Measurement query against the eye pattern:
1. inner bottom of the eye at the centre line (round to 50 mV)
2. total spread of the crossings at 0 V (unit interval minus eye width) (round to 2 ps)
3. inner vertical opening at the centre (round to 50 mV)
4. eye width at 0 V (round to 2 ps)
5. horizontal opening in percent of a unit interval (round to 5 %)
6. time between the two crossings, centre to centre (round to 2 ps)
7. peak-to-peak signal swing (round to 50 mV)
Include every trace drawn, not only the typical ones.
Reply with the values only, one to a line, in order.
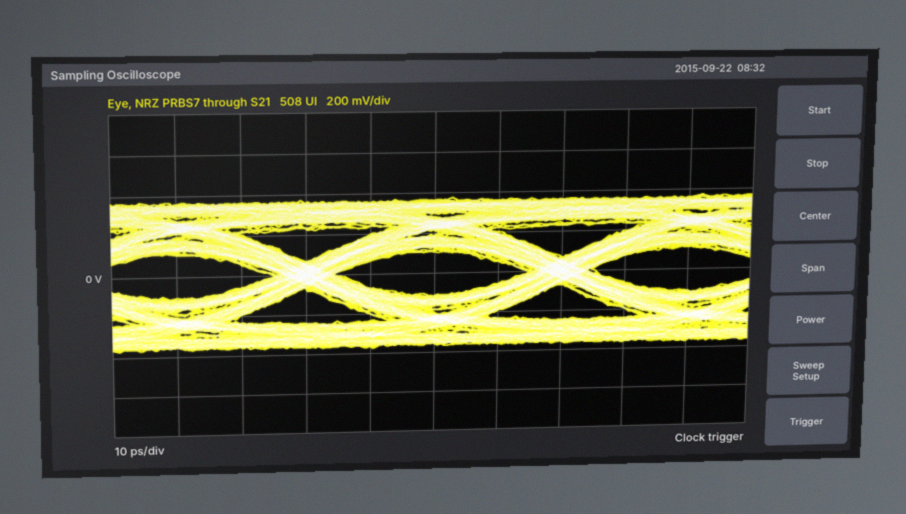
-100 mV
10 ps
200 mV
30 ps
75 %
40 ps
750 mV
